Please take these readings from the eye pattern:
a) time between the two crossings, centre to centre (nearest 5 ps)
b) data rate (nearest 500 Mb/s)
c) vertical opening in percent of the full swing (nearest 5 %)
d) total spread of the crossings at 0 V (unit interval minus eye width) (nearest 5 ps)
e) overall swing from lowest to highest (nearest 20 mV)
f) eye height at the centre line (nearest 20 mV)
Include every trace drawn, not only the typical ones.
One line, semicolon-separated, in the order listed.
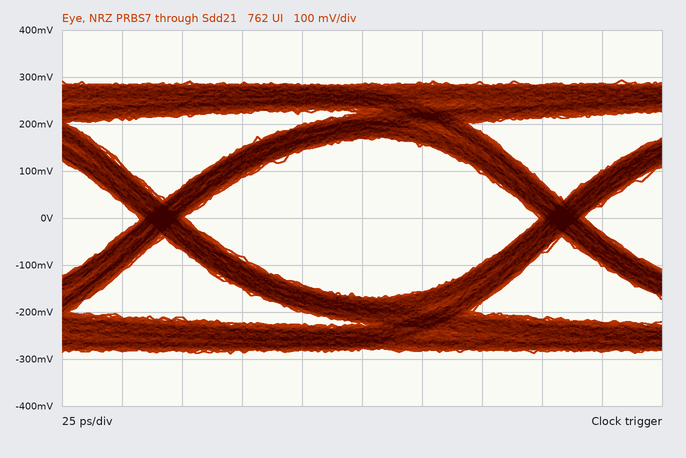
165 ps; 6.0 Gb/s; 60 %; 20 ps; 580 mV; 340 mV
